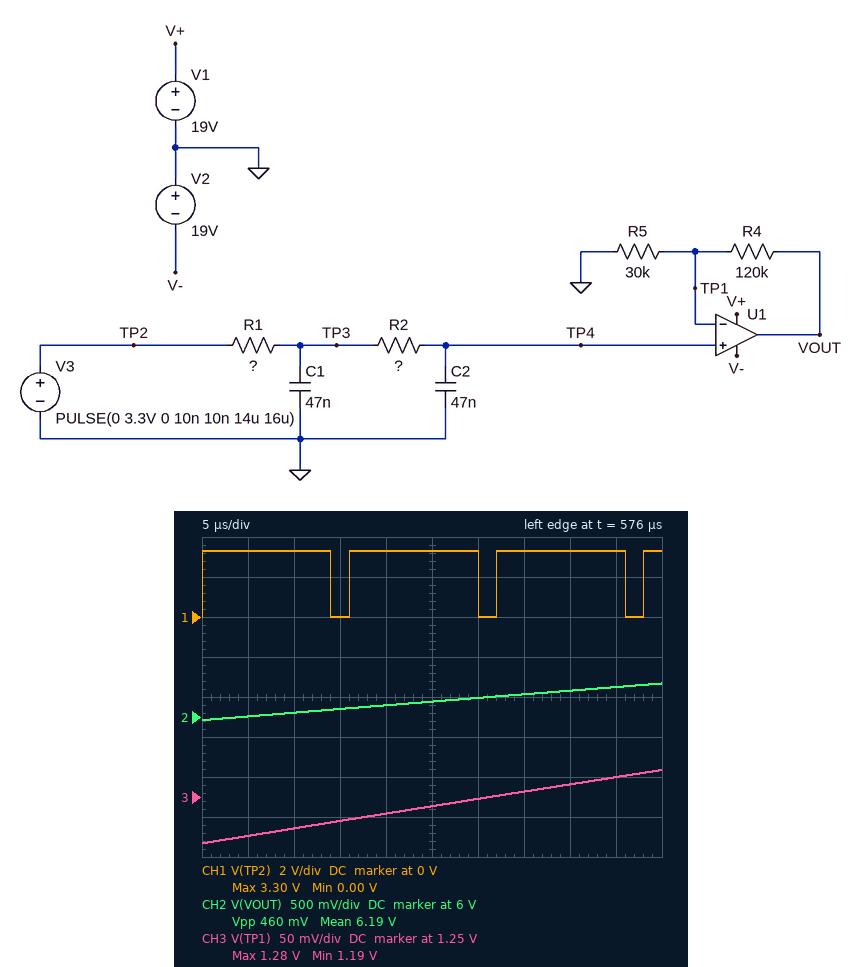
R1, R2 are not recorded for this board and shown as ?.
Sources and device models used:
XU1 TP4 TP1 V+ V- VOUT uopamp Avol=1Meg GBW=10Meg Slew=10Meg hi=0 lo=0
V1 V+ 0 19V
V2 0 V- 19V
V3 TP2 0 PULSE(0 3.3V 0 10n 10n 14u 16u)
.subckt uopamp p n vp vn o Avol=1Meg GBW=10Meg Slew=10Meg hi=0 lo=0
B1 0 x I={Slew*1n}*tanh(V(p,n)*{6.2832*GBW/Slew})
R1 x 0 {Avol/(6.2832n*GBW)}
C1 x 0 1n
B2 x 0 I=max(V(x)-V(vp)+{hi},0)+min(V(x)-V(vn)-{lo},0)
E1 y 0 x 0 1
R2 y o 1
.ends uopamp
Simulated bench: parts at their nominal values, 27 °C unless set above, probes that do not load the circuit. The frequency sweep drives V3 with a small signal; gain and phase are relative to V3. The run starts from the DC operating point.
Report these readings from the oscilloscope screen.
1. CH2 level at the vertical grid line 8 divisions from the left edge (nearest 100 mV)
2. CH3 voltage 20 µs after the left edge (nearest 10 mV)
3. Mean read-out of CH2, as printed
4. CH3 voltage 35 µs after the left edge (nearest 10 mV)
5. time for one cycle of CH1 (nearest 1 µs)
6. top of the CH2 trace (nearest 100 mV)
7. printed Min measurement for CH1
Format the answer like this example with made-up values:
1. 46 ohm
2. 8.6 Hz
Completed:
1. 6.3 V
2. 1.23 V
3. 6.19 V
4. 1.26 V
5. 16 µs
6. 6.4 V
7. 0.00 V
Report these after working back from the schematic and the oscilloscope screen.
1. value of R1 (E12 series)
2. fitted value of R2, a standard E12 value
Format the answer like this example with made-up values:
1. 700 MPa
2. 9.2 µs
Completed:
1. 8.2 kΩ
2. 4.7 kΩ
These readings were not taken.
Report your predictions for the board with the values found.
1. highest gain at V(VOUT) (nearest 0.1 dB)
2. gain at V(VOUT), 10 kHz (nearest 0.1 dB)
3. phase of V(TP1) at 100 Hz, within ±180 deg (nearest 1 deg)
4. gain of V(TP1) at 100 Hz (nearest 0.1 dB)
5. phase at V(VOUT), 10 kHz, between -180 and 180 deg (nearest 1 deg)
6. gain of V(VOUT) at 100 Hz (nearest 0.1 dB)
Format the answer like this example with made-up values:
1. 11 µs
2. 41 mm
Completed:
1. 14.0 dB
2. -36.7 dB
3. -33 deg
4. -1.2 dB
5. -170 deg
6. 12.8 dB
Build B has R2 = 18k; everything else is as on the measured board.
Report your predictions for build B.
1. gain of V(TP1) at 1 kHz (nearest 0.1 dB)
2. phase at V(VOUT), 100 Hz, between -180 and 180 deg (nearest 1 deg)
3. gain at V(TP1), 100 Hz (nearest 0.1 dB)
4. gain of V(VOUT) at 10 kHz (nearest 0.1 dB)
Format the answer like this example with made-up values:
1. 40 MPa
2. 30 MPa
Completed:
1. -23.9 dB
2. -49 deg
3. -2.5 dB
4. -48.2 dB
